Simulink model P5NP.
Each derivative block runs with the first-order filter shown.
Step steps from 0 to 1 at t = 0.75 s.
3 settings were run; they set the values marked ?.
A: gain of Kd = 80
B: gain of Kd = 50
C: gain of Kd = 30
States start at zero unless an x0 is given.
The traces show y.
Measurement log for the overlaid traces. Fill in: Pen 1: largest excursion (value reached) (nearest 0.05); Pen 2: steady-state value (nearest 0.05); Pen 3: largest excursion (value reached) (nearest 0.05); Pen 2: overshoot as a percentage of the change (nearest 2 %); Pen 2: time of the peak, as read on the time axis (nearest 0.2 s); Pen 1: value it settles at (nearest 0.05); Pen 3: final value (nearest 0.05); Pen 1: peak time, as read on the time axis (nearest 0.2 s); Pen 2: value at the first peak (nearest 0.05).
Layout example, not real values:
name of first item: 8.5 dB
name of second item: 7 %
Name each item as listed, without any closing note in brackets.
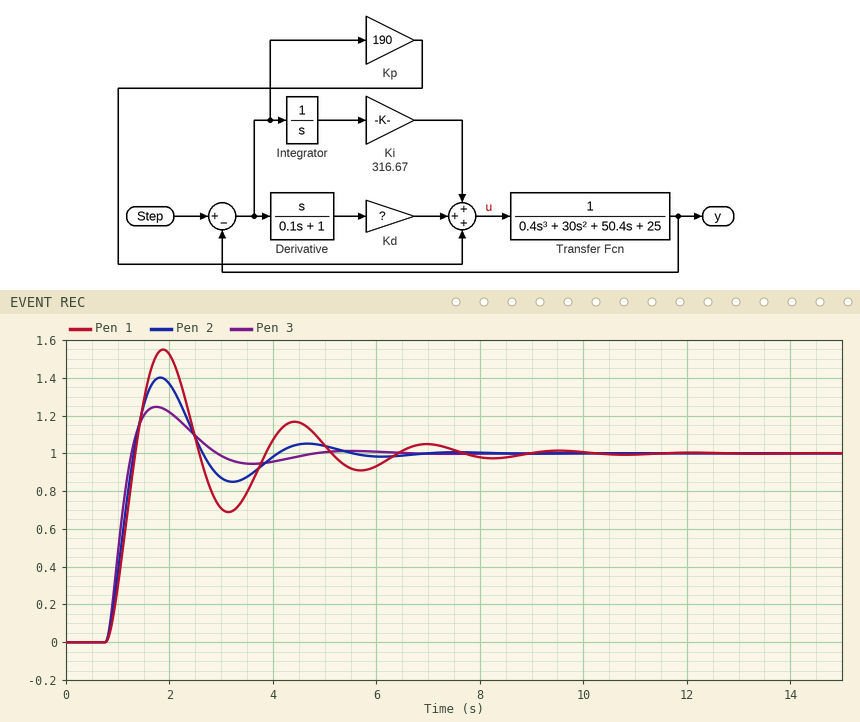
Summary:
Pen 1: largest excursion (value reached): 1.55
Pen 2: steady-state value: 1.00
Pen 3: largest excursion (value reached): 1.25
Pen 2: overshoot as a percentage of the change: 40 %
Pen 2: time of the peak, as read on the time axis: 1.8 s
Pen 1: value it settles at: 1.00
Pen 3: final value: 1.00
Pen 1: peak time, as read on the time axis: 1.8 s
Pen 2: value at the first peak: 1.40
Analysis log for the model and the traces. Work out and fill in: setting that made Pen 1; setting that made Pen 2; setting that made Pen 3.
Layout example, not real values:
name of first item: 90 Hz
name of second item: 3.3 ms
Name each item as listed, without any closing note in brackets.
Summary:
setting that made Pen 1: C
setting that made Pen 2: B
setting that made Pen 3: A
